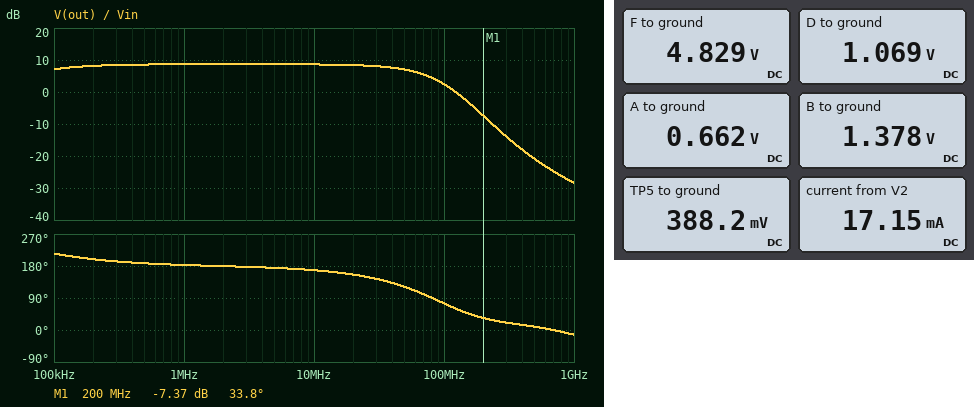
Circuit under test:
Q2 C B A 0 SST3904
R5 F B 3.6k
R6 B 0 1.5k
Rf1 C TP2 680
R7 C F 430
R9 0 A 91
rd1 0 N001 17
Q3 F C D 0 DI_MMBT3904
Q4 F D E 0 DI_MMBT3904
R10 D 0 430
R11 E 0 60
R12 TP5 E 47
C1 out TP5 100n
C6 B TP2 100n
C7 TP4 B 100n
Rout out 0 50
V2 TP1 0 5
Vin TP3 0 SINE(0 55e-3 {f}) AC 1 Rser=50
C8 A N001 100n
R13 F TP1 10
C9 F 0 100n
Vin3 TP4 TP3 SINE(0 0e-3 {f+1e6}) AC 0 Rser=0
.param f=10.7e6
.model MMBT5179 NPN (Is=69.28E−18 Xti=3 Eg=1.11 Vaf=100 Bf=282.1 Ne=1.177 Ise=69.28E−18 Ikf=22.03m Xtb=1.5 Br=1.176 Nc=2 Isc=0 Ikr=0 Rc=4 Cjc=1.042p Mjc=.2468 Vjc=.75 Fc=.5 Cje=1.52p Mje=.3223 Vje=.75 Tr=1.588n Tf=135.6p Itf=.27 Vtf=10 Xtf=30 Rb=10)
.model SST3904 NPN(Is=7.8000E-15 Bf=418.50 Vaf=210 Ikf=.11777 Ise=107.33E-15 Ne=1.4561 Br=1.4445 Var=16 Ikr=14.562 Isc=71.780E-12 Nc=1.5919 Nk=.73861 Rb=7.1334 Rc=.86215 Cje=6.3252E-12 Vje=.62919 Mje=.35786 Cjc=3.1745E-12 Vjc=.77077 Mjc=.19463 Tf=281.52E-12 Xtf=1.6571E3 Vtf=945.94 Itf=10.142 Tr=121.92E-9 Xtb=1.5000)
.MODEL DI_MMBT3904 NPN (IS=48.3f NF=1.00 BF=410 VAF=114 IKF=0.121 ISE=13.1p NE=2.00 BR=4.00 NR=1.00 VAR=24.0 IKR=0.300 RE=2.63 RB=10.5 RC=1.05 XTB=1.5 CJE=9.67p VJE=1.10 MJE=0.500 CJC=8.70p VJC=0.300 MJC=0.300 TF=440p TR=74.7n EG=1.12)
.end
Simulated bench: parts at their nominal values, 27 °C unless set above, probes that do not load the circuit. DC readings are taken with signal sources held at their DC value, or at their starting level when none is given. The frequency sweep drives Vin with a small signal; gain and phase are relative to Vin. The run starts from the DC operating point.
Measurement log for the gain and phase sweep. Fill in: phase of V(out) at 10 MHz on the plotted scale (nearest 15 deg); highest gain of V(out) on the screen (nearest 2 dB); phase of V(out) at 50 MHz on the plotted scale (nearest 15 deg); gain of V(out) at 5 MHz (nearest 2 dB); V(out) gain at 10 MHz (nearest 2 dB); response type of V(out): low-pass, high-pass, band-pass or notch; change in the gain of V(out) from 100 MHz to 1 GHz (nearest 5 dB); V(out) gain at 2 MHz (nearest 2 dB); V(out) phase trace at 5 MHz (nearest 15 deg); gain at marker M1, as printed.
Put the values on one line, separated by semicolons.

165 deg; 8 dB; 120 deg; 8 dB; 8 dB; low-pass; -30 dB; 8 dB; 180 deg; -7.37 dB
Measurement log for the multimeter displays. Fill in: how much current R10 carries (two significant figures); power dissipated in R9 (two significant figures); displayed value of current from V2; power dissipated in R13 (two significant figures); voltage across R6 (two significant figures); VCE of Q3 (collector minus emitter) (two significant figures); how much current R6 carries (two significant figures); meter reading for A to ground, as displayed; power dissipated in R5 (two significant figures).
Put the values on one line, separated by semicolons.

2.5 mA; 4.8 mW; 17.15 mA; 2.9 mW; 1.4 V; 3.8 V; 920 µA; 0.662 V; 3.3 mW
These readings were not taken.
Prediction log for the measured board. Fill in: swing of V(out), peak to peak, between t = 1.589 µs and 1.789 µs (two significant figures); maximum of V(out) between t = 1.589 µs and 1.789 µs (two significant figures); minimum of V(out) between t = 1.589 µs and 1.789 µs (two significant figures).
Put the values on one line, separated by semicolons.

270 mV; 150 mV; -120 mV
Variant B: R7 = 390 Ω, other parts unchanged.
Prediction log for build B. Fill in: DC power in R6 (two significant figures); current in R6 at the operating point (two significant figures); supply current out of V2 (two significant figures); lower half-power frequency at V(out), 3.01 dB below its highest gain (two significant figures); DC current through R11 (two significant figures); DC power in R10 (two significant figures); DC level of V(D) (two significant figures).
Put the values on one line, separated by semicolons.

1.2 mW; 910 µA; 22 mA; 67 kHz; 11 mA; 4.3 mW; 1.4 V
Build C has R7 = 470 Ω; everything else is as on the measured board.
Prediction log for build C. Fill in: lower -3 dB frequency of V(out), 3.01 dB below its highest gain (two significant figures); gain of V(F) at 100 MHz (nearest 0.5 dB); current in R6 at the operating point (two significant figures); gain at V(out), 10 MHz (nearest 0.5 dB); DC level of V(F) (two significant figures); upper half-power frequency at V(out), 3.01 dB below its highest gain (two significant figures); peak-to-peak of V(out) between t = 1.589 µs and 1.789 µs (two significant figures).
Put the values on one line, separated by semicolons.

63 kHz; -59.5 dB; 930 µA; 7.5 dB; 4.9 V; 63 MHz; 190 mV
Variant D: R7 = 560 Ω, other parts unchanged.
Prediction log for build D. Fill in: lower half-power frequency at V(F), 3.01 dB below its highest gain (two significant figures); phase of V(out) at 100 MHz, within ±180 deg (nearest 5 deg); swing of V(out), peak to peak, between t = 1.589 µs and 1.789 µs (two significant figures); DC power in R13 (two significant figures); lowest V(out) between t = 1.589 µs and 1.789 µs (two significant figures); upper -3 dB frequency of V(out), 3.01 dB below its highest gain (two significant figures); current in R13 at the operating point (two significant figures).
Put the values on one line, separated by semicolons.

30 kHz; 125 deg; 18 mV; 780 µW; -4.8 mV; 190 MHz; 8.8 mA
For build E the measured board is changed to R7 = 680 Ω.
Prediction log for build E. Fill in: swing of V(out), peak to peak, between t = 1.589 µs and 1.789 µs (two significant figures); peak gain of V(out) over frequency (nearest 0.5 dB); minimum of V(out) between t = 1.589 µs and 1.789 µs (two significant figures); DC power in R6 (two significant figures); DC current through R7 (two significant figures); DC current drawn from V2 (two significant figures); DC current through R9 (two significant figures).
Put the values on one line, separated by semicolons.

9.6 mV; -29.0 dB; -3.3 mV; 1.1 mW; 6.2 mA; 7.5 mA; 6.3 mA
